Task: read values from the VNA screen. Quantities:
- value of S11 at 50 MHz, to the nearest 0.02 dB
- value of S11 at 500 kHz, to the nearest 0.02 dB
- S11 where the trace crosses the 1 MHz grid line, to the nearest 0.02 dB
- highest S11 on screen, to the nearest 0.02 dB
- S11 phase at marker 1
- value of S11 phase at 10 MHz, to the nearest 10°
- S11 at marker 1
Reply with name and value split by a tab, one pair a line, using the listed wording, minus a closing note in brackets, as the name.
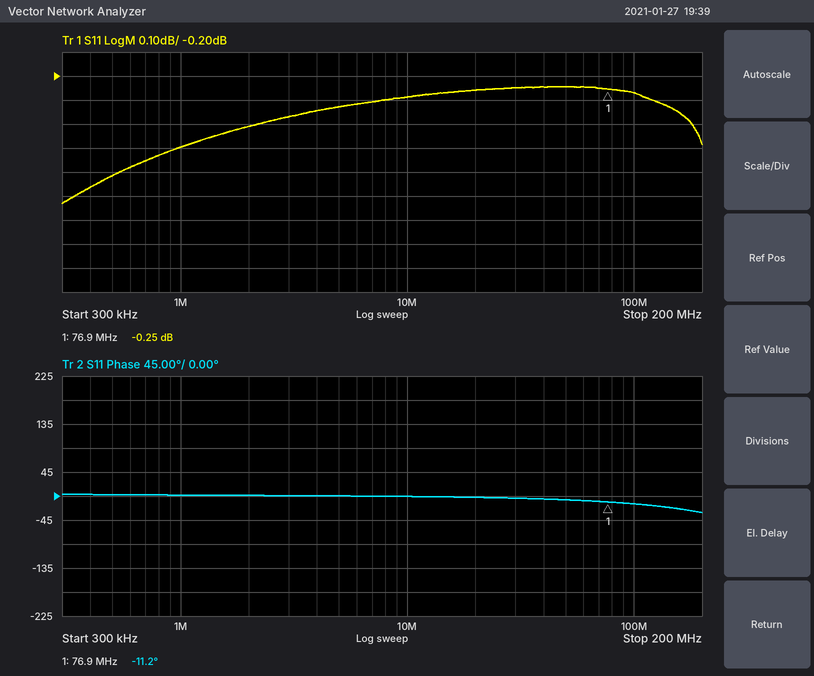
value of S11 at 50 MHz, to the nearest 0.02 dB	-0.24 dB
value of S11 at 500 kHz, to the nearest 0.02 dB	-0.62 dB
S11 where the trace crosses the 1 MHz grid line, to the nearest 0.02 dB	-0.50 dB
highest S11 on screen, to the nearest 0.02 dB	-0.24 dB
S11 phase at marker 1	-11.2°
value of S11 phase at 10 MHz, to the nearest 10°	0°
S11 at marker 1	-0.25 dB
